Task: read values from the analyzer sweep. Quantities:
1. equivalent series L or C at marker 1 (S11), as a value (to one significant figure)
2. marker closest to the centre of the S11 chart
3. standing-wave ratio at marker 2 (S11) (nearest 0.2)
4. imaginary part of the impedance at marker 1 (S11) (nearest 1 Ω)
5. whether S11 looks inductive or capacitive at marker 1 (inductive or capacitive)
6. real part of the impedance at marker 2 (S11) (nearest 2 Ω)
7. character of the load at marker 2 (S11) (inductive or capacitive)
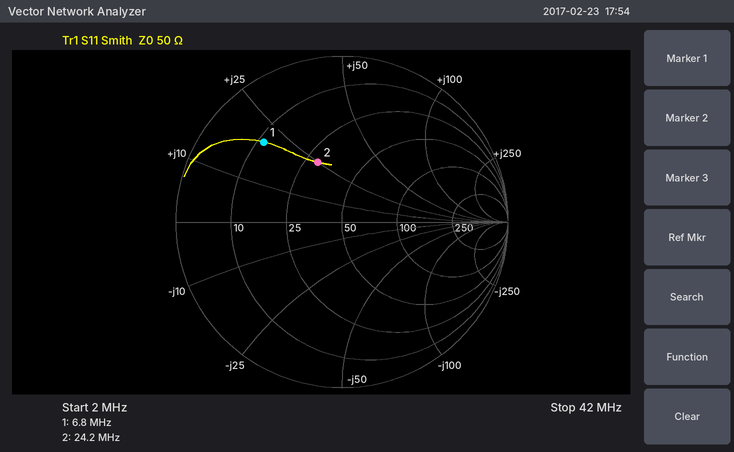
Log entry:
500 nH
marker 2
2.2
+20 Ω
inductive
30 Ω
inductive
